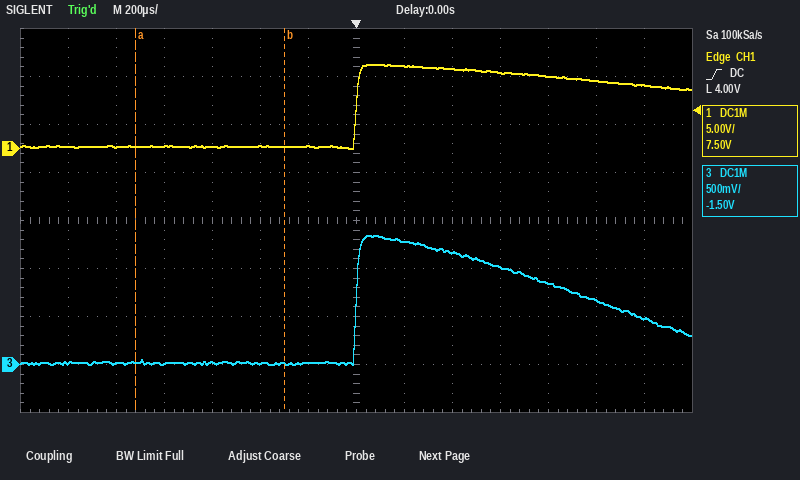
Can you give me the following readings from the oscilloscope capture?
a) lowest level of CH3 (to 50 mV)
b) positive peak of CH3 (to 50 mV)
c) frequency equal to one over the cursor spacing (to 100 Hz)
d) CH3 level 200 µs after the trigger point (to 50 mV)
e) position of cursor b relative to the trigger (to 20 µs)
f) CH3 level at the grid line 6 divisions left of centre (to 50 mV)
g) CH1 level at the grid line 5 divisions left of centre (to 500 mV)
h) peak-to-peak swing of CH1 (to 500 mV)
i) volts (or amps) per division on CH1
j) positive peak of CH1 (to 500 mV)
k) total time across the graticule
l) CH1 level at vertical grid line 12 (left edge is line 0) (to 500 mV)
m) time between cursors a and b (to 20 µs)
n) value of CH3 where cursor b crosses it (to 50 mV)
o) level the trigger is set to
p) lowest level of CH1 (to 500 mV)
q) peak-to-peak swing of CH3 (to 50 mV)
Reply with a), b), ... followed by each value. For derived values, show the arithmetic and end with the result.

a) 0 mV
b) 1.35 V
c) 1 / 620 µs ≈ 1.6 kHz
d) 1.30 V
e) -300 µs
f) 0 mV
g) 0.0 V
h) 9.0 V − (0.0 V) = 9.0 V
i) 5 V
j) 9.0 V
k) 2.8 ms
l) 7.0 V
m) 620 µs
n) 0 mV
o) 4.00 V
p) 0.0 V
q) 1.35 V − (0 mV) = 1.35 V
